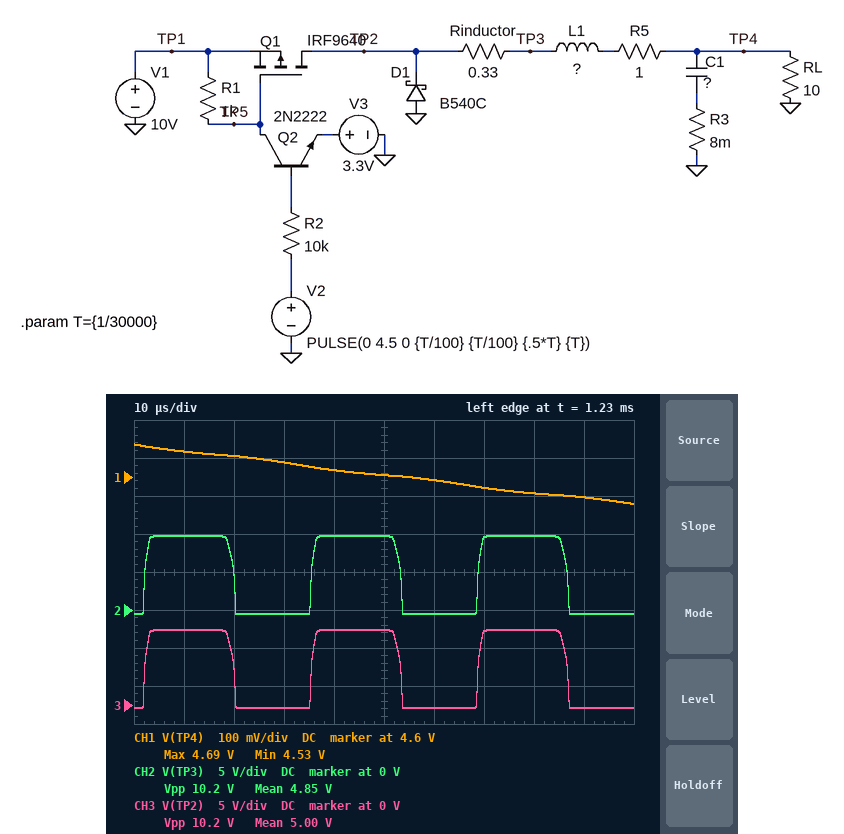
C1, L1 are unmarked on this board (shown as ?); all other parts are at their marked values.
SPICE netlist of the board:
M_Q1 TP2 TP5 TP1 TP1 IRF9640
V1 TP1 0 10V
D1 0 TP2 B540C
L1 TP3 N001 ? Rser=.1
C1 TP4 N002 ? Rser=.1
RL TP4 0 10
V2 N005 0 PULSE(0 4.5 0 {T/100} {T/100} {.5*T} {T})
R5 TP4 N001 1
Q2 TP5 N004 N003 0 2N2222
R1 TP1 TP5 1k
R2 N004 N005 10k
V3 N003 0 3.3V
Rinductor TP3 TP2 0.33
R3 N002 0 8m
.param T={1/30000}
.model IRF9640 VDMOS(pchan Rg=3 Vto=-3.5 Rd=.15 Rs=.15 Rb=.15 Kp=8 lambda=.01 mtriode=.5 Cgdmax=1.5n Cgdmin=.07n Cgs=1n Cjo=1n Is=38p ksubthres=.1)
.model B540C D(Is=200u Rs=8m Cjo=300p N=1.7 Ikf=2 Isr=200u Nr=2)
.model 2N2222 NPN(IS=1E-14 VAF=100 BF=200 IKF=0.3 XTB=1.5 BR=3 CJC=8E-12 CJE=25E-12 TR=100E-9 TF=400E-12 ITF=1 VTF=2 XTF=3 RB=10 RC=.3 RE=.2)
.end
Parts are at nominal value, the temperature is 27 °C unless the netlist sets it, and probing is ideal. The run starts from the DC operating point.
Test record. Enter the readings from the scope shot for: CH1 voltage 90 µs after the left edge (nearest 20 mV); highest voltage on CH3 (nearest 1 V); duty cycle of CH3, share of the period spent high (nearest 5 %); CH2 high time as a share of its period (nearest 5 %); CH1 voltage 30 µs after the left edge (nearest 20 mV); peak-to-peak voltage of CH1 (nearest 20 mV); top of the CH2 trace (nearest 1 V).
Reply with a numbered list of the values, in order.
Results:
1. 4.54 V
2. 10 V
3. 55 %
4. 55 %
5. 4.64 V
6. 160 mV
7. 10 V
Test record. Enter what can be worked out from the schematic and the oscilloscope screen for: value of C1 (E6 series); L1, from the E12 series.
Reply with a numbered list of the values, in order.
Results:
1. 33 µF
2. 2.2 mH
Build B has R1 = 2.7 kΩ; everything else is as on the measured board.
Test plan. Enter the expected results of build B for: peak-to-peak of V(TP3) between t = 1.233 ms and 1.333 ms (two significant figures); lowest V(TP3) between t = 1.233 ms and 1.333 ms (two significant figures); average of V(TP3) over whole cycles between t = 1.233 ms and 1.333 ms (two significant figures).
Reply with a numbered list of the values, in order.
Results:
1. 10 V
2. -540 mV
3. 6.2 V
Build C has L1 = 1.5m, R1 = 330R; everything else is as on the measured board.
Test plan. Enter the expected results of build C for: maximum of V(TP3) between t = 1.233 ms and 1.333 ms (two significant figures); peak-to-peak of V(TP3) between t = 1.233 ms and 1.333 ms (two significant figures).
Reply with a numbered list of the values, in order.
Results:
1. 250 mV
2. 290 mV
